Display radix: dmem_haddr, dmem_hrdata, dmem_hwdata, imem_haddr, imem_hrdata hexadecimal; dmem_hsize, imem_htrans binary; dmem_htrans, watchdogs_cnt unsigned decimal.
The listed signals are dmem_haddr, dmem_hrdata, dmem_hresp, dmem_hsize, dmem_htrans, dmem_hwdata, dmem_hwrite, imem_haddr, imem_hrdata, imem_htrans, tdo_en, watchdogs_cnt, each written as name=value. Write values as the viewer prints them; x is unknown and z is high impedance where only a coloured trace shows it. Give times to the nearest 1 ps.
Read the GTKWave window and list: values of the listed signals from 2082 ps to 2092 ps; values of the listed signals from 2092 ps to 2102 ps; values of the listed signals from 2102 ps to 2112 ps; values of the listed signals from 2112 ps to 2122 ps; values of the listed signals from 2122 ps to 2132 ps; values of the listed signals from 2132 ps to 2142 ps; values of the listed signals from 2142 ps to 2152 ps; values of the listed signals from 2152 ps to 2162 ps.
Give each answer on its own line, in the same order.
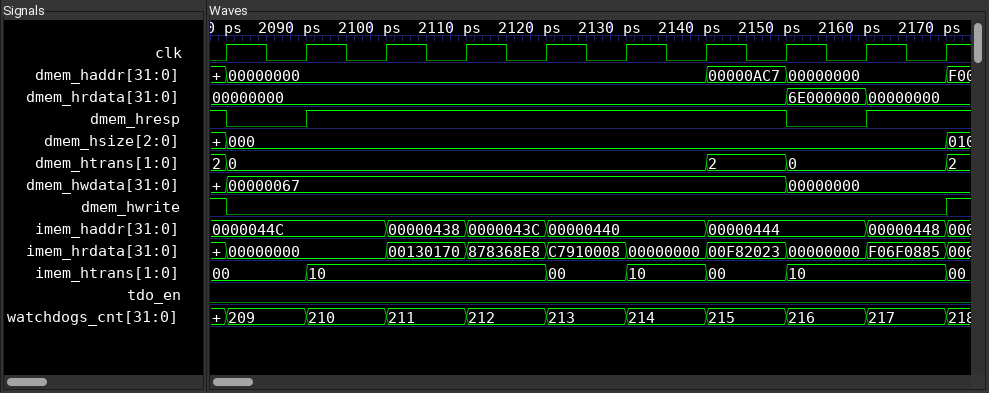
dmem_haddr=00000000, dmem_hrdata=00000000, dmem_hresp=0, dmem_hsize=000, dmem_htrans=0, dmem_hwdata=00000067, dmem_hwrite=0, imem_haddr=0000044C, imem_hrdata=00000000, imem_htrans=00, tdo_en=0, watchdogs_cnt=209
dmem_haddr=00000000, dmem_hrdata=00000000, dmem_hresp=1, dmem_hsize=000, dmem_htrans=0, dmem_hwdata=00000067, dmem_hwrite=0, imem_haddr=0000044C, imem_hrdata=00000000, imem_htrans=10, tdo_en=0, watchdogs_cnt=210
dmem_haddr=00000000, dmem_hrdata=00000000, dmem_hresp=1, dmem_hsize=000, dmem_htrans=0, dmem_hwdata=00000067, dmem_hwrite=0, imem_haddr=00000438, imem_hrdata=00130170, imem_htrans=10, tdo_en=0, watchdogs_cnt=211
dmem_haddr=00000000, dmem_hrdata=00000000, dmem_hresp=1, dmem_hsize=000, dmem_htrans=0, dmem_hwdata=00000067, dmem_hwrite=0, imem_haddr=0000043C, imem_hrdata=878368E8, imem_htrans=10, tdo_en=0, watchdogs_cnt=212
dmem_haddr=00000000, dmem_hrdata=00000000, dmem_hresp=1, dmem_hsize=000, dmem_htrans=0, dmem_hwdata=00000067, dmem_hwrite=0, imem_haddr=00000440, imem_hrdata=C7910008, imem_htrans=00, tdo_en=0, watchdogs_cnt=213
dmem_haddr=00000000, dmem_hrdata=00000000, dmem_hresp=1, dmem_hsize=000, dmem_htrans=0, dmem_hwdata=00000067, dmem_hwrite=0, imem_haddr=00000440, imem_hrdata=00000000, imem_htrans=10, tdo_en=0, watchdogs_cnt=214
dmem_haddr=00000AC7, dmem_hrdata=00000000, dmem_hresp=1, dmem_hsize=000, dmem_htrans=2, dmem_hwdata=00000067, dmem_hwrite=0, imem_haddr=00000444, imem_hrdata=00F82023, imem_htrans=00, tdo_en=0, watchdogs_cnt=215
dmem_haddr=00000000, dmem_hrdata=6E000000, dmem_hresp=0, dmem_hsize=000, dmem_htrans=0, dmem_hwdata=00000000, dmem_hwrite=0, imem_haddr=00000444, imem_hrdata=00000000, imem_htrans=10, tdo_en=0, watchdogs_cnt=216
